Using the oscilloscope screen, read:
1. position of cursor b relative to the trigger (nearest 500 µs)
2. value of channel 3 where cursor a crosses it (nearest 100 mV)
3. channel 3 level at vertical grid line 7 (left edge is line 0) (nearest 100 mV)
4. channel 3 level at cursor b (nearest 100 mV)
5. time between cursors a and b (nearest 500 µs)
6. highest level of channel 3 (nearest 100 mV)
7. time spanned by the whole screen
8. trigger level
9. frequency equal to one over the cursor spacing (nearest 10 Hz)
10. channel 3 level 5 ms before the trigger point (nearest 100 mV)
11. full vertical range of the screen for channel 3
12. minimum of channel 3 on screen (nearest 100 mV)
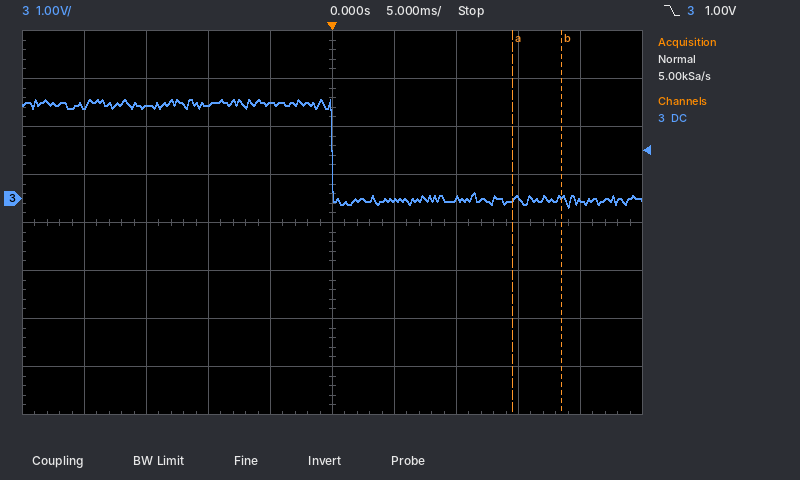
+18.5 ms
0.0 V
0.0 V
0.0 V
4.0 ms
2.1 V
50 ms
1.00 V
250 Hz
2.0 V
8 V
-200 mV
